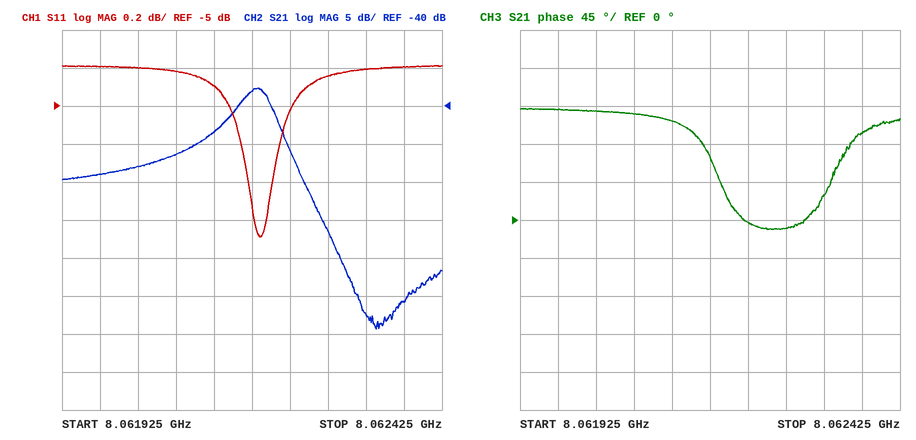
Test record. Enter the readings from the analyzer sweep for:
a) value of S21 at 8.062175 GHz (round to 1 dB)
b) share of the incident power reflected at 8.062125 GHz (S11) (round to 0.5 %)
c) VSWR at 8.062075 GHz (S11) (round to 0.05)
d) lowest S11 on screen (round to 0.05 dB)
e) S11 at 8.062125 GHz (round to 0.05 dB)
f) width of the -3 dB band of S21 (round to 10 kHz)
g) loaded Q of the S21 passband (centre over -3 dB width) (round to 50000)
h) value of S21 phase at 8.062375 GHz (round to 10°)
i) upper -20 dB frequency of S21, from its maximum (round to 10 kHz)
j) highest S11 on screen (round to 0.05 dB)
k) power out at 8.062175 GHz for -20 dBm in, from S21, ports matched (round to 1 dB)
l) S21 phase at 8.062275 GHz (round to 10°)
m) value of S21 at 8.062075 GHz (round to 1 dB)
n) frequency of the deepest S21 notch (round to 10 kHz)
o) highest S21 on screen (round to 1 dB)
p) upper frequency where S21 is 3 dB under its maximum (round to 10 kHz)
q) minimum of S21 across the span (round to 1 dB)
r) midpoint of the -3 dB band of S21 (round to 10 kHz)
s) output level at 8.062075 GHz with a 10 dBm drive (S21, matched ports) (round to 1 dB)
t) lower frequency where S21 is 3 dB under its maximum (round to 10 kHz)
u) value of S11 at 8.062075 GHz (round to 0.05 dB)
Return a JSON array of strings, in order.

["-38 dB", "32.5 %", "3.70", "-5.70 dB", "-4.90 dB", "50 kHz", "150000", "100°", "8.06228 GHz", "-4.80 dB", "-58 dBm", "-10°", "-46 dB", "8.06234 GHz", "-38 dB", "8.06220 GHz", "-69 dB", "8.06218 GHz", "-36 dBm", "8.06215 GHz", "-4.80 dB"]
